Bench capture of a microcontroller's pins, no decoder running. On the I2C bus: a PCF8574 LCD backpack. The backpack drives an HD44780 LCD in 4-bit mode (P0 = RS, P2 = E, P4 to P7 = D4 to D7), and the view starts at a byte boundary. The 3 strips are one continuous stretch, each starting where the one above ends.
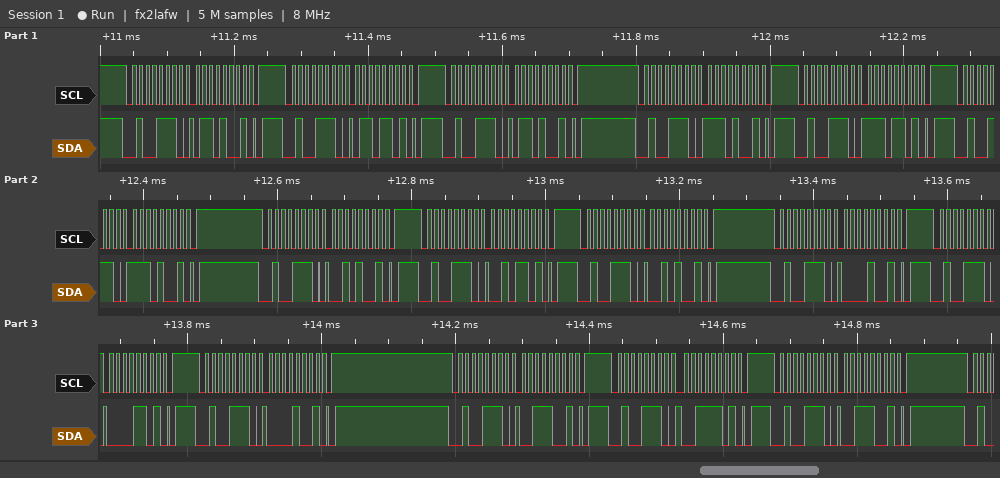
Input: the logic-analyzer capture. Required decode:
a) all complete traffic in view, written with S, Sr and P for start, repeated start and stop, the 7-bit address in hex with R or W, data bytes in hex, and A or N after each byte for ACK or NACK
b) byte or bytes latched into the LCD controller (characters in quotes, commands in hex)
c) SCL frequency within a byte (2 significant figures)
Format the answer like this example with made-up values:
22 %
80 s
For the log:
S 27W A 69 A P S 27W A 6D A P S 27W A 69 A P S 27W A E9 A P S 27W A ED A P S 27W A E9 A P S 27W A 29 A P S 27W A 2D A P S 27W A 29 A P S 27W A 09 A P S 27W A 0D A P S 27W A 09 A P S 27W A 39 A P S 27W A 3D A P S 27W A 39 A P
'n' ' '
100 kHz
